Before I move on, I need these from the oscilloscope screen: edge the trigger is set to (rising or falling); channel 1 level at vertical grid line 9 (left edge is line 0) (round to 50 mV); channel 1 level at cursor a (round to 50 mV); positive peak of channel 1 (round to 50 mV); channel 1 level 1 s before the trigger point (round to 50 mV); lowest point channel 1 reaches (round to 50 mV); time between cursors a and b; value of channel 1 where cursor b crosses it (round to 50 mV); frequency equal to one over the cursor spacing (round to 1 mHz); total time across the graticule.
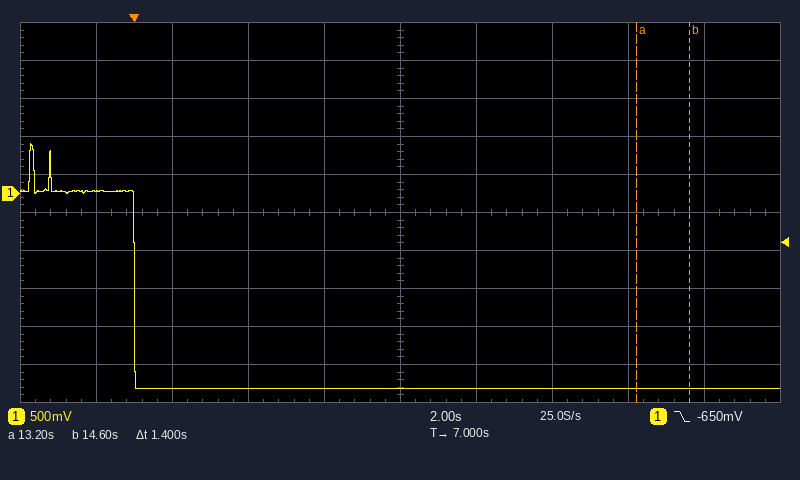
falling
-2.55 V
-2.55 V
650 mV
50 mV
-2.55 V
1.4 s
-2.55 V
714 mHz
20 s
